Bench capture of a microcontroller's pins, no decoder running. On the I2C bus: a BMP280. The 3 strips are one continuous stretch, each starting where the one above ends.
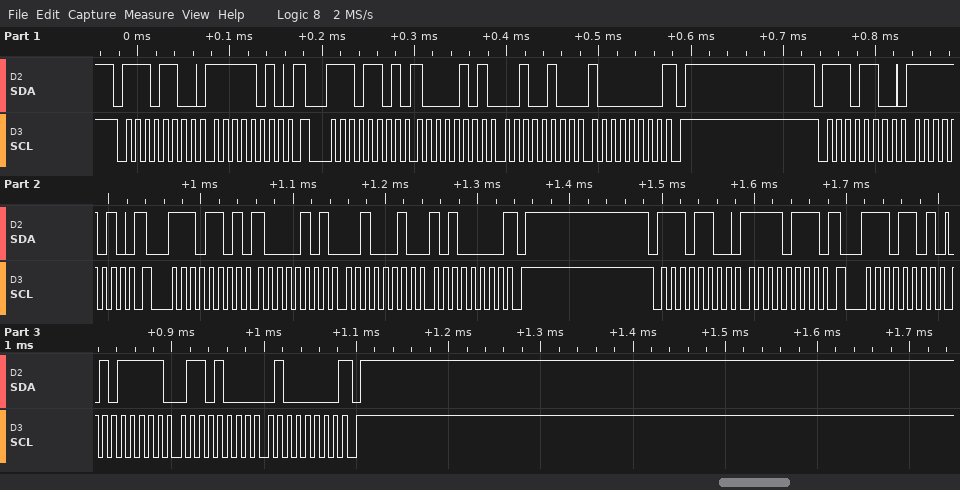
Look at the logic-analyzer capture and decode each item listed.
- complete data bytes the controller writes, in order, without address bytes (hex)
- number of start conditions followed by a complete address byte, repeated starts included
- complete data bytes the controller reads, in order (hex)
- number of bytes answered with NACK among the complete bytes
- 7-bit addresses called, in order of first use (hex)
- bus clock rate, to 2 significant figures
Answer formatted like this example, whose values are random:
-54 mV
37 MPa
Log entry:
FA FA F7
6
85 24 80 85 22 A0 5F 68 40
3
0x76
100 kHz
